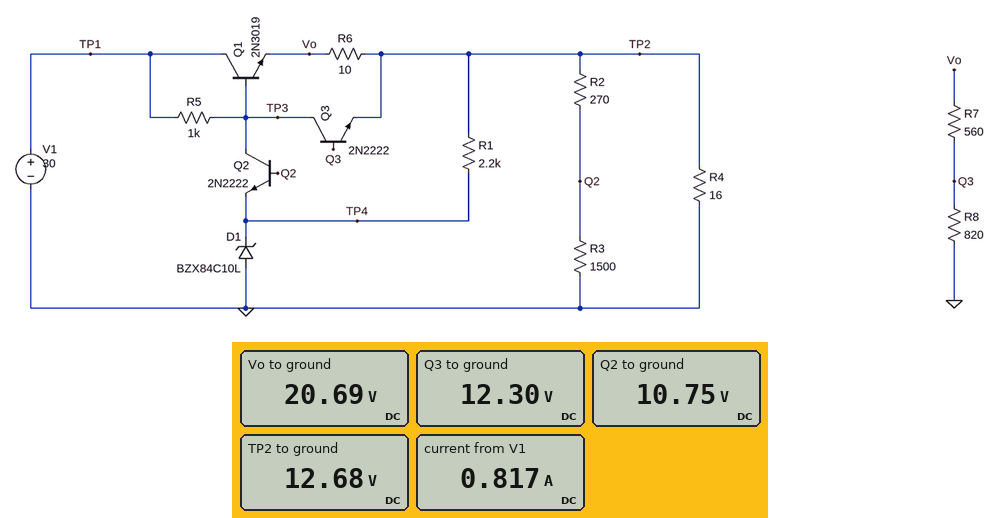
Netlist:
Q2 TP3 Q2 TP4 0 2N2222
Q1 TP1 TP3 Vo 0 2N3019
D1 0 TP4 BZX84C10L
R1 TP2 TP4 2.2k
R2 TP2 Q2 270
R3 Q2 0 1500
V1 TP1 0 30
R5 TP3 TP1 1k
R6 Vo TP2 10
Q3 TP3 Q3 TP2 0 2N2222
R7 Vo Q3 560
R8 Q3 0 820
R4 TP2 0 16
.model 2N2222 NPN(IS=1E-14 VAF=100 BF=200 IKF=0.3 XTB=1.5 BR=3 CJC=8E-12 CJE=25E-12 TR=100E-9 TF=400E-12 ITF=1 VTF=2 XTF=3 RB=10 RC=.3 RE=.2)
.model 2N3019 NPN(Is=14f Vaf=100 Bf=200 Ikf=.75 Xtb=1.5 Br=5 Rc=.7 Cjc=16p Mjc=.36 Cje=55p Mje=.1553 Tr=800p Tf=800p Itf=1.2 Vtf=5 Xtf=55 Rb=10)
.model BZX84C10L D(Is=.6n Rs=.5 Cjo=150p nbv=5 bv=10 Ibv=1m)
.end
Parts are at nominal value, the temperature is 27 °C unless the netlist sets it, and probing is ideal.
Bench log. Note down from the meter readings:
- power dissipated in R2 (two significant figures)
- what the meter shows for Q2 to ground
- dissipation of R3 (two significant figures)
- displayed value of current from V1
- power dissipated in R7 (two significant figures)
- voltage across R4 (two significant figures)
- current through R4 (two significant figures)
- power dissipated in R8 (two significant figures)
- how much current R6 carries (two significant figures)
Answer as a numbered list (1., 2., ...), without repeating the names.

1. 14 mW
2. 10.75 V
3. 77 mW
4. 0.817 A
5. 130 mW
6. 13 V
7. 790 mA
8. 180 mW
9. 800 mA
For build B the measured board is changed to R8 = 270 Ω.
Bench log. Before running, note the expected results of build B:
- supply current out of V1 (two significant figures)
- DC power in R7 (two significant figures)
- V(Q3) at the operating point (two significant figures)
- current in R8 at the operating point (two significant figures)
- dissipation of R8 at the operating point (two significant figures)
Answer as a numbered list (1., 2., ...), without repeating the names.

1. 830 mA
2. 350 mW
3. 6.7 V
4. 25 mA
5. 170 mW
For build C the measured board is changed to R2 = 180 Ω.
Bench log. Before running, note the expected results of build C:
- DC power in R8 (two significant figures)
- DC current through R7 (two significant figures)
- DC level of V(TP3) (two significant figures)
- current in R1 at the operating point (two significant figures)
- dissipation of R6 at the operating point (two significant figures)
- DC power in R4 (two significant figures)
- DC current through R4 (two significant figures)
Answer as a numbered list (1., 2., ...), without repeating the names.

1. 170 mW
2. 14 mA
3. 21 V
4. 900 µA
5. 5.9 W
6. 9.2 W
7. 760 mA
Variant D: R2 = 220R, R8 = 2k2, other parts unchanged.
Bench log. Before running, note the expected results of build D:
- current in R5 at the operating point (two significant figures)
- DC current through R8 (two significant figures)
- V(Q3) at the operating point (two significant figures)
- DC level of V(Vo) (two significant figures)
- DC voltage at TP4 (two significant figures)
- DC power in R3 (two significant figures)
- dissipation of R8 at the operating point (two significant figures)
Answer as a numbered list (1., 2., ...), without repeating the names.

1. 24 mA
2. 1.8 mA
3. 4.0 V
4. 5.1 V
5. 3.3 V
6. 5.5 mW
7. 7.4 mW
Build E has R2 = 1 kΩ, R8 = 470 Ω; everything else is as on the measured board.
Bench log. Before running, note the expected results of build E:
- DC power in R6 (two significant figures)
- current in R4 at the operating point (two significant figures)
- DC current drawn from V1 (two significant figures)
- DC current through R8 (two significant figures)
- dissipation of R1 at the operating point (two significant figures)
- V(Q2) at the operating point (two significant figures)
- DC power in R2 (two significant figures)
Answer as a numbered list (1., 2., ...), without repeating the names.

1. 6.7 W
2. 810 mA
3. 840 mA
4. 21 mA
5. 4.0 mW
6. 7.8 V
7. 27 mW
